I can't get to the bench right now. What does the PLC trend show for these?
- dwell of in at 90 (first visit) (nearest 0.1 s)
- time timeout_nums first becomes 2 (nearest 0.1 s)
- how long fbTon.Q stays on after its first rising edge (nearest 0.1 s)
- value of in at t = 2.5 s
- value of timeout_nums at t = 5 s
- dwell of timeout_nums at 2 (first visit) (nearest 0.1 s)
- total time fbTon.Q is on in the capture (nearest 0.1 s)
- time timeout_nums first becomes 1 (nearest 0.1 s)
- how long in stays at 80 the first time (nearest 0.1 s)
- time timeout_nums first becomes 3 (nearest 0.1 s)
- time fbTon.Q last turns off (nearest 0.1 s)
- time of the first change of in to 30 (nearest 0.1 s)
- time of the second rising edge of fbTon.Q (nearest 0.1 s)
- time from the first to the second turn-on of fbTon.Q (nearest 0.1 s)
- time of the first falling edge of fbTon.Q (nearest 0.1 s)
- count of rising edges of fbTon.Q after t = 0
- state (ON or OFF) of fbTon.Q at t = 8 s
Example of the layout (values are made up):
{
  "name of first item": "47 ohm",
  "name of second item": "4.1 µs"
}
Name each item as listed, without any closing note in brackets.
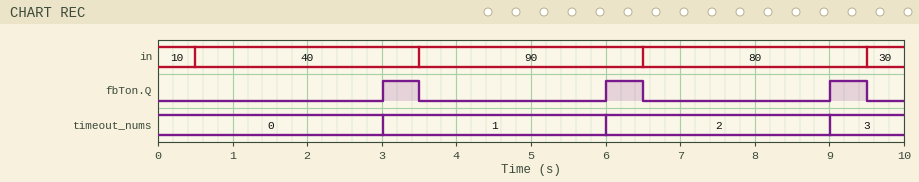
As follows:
{
  "dwell of in at 90 (first visit)": "3.0 s",
  "time timeout_nums first becomes 2": "6.0 s",
  "how long fbTon.Q stays on after its first rising edge": "0.5 s",
  "value of in at t = 2.5 s": "40",
  "value of timeout_nums at t = 5 s": "1",
  "dwell of timeout_nums at 2 (first visit)": "3.0 s",
  "total time fbTon.Q is on in the capture": "1.5 s",
  "time timeout_nums first becomes 1": "3.0 s",
  "how long in stays at 80 the first time": "3.0 s",
  "time timeout_nums first becomes 3": "9.0 s",
  "time fbTon.Q last turns off": "9.5 s",
  "time of the first change of in to 30": "9.5 s",
  "time of the second rising edge of fbTon.Q": "6.0 s",
  "time from the first to the second turn-on of fbTon.Q": "3.0 s",
  "time of the first falling edge of fbTon.Q": "3.5 s",
  "count of rising edges of fbTon.Q after t = 0": "3",
  "state (ON or OFF) of fbTon.Q at t = 8 s": "OFF"
}
